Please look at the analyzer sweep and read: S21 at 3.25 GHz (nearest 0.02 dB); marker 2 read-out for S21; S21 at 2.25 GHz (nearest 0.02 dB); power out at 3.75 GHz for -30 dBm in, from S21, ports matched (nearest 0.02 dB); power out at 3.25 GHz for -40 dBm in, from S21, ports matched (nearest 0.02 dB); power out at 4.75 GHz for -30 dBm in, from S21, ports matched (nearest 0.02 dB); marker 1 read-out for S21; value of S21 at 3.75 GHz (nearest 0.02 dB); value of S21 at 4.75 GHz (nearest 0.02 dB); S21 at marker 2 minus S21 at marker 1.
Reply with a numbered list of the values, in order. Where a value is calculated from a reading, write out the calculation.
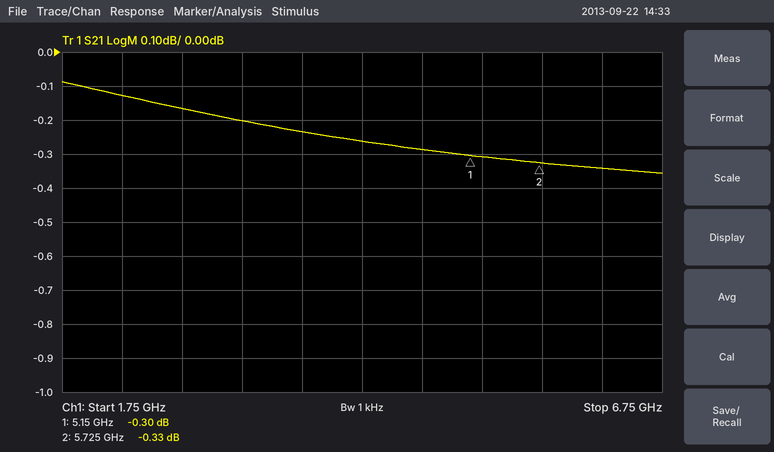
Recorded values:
1. -0.20 dB
2. -0.33 dB
3. -0.12 dB
4. -30 dBm + (-0.24 dB) = -30.24 dBm
5. -40 dBm + (-0.20 dB) = -40.20 dBm
6. -30 dBm + (-0.28 dB) = -30.28 dBm
7. -0.30 dB
8. -0.24 dB
9. -0.28 dB
10. -0.33 − (-0.3) = -0.03 dB
